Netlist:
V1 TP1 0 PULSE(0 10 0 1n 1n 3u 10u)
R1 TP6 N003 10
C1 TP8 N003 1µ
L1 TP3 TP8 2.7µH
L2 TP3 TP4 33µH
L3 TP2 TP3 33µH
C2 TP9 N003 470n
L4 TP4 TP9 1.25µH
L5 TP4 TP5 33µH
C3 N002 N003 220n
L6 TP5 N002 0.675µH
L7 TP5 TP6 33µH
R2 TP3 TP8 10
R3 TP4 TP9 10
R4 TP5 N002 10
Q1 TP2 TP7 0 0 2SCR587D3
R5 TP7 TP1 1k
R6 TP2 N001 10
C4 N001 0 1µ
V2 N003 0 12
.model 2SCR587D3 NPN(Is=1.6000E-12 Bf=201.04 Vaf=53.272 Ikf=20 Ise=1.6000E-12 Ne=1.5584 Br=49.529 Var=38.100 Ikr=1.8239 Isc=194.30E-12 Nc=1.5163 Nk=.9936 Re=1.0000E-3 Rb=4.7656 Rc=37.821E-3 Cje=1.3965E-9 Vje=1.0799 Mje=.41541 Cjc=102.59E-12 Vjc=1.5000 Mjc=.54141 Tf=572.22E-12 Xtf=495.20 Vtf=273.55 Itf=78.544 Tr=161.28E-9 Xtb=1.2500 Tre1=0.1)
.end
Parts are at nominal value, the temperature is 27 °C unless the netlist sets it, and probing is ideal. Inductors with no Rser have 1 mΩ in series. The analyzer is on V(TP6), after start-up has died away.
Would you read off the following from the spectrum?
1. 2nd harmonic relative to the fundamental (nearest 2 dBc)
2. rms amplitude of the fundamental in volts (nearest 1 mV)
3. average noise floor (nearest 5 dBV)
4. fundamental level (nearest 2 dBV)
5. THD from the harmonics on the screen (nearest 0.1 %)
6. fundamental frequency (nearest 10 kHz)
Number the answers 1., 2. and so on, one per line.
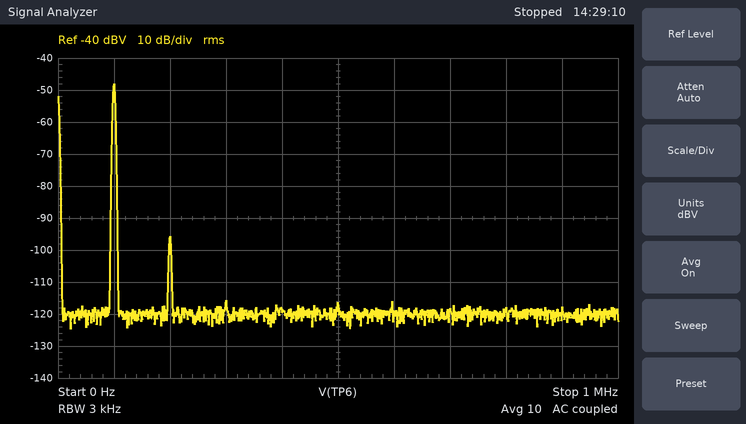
1. -48 dBc
2. 4 mV
3. -120 dBV
4. -48 dBV
5. 0.4 %
6. 100 kHz
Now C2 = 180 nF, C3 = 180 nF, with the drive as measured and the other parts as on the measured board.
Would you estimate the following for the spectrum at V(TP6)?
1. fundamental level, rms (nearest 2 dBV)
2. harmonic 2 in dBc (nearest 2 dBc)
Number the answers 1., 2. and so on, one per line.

1. -28 dBV
2. -44 dBc
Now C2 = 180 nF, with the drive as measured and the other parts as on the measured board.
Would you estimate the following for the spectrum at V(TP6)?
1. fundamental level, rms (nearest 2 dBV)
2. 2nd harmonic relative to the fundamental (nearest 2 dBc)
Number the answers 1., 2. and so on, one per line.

1. -24 dBV
2. -50 dBc
